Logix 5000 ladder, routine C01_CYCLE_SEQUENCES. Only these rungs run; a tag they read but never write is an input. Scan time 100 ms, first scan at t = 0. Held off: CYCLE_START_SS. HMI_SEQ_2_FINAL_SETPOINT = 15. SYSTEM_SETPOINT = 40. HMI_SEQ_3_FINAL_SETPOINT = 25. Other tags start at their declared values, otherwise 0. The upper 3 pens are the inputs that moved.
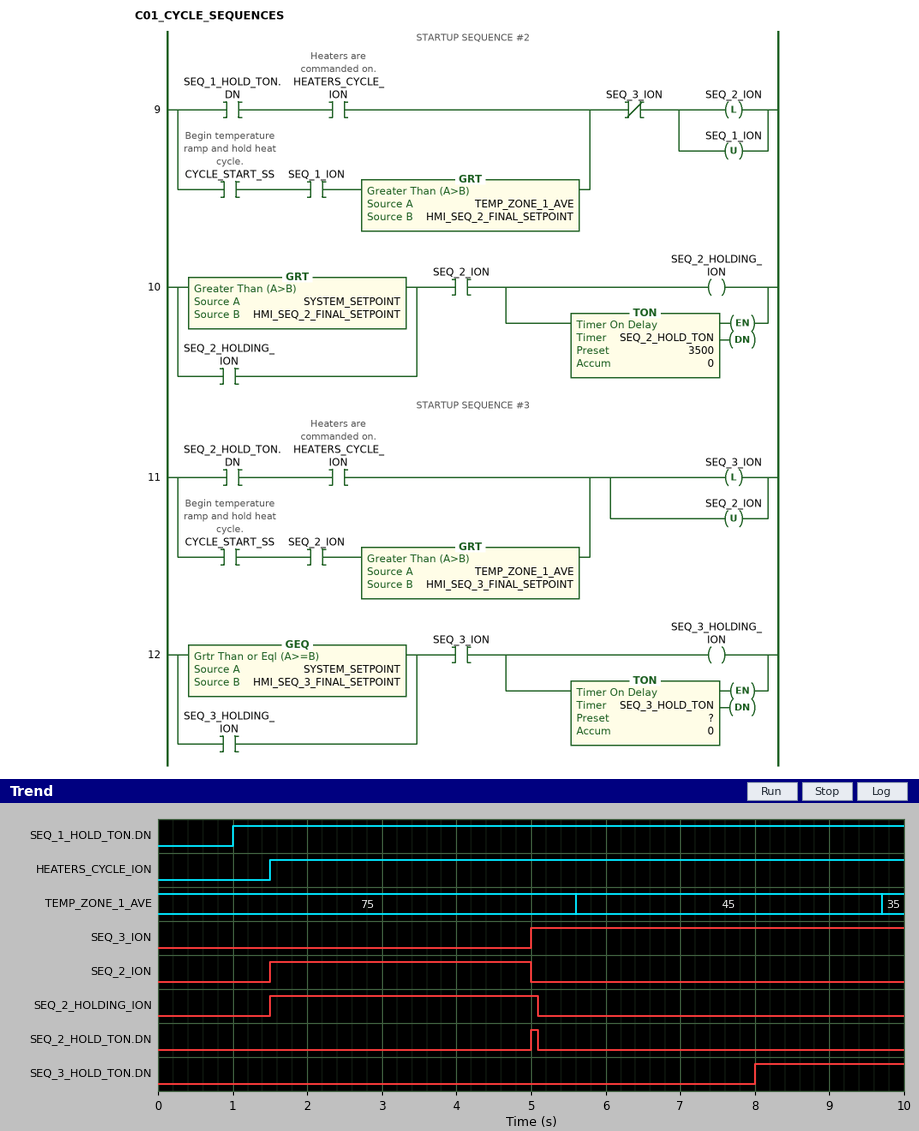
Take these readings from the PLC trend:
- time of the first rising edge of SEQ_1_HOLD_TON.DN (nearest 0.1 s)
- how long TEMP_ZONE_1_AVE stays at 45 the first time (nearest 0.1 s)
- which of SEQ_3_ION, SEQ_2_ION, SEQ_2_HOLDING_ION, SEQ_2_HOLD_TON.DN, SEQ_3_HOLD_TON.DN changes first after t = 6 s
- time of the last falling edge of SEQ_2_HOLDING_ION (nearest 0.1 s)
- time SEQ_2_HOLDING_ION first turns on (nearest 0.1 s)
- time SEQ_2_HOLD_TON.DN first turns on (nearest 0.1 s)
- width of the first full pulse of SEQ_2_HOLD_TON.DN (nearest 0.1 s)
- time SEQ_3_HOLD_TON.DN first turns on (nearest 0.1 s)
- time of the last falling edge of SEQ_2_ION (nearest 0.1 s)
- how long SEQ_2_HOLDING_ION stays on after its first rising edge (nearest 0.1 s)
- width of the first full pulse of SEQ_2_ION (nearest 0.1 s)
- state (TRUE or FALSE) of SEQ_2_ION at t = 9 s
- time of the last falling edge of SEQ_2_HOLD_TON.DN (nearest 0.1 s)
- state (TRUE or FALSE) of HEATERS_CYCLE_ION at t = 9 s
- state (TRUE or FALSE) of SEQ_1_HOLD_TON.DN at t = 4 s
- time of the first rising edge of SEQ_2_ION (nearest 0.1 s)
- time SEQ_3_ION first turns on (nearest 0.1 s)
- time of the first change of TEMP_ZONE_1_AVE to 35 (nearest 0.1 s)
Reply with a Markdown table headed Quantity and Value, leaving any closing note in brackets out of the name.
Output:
| Quantity | Value |
|---|---|
| time of the first rising edge of SEQ_1_HOLD_TON.DN | 1.0 s |
| how long TEMP_ZONE_1_AVE stays at 45 the first time | 4.1 s |
| which of SEQ_3_ION, SEQ_2_ION, SEQ_2_HOLDING_ION, SEQ_2_HOLD_TON.DN, SEQ_3_HOLD_TON.DN changes first after t = 6 s | SEQ_3_HOLD_TON.DN |
| time of the last falling edge of SEQ_2_HOLDING_ION | 5.1 s |
| time SEQ_2_HOLDING_ION first turns on | 1.5 s |
| time SEQ_2_HOLD_TON.DN first turns on | 5.0 s |
| width of the first full pulse of SEQ_2_HOLD_TON.DN | 0.1 s |
| time SEQ_3_HOLD_TON.DN first turns on | 8.0 s |
| time of the last falling edge of SEQ_2_ION | 5.0 s |
| how long SEQ_2_HOLDING_ION stays on after its first rising edge | 3.6 s |
| width of the first full pulse of SEQ_2_ION | 3.5 s |
| state (TRUE or FALSE) of SEQ_2_ION at t = 9 s | FALSE |
| time of the last falling edge of SEQ_2_HOLD_TON.DN | 5.1 s |
| state (TRUE or FALSE) of HEATERS_CYCLE_ION at t = 9 s | TRUE |
| state (TRUE or FALSE) of SEQ_1_HOLD_TON.DN at t = 4 s | TRUE |
| time of the first rising edge of SEQ_2_ION | 1.5 s |
| time SEQ_3_ION first turns on | 5.0 s |
| time of the first change of TEMP_ZONE_1_AVE to 35 | 9.7 s |
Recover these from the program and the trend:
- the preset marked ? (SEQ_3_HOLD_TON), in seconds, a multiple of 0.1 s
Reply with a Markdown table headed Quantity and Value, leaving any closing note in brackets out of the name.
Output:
| Quantity | Value |
|---|---|
| the preset marked ? (SEQ_3_HOLD_TON), in seconds, a multiple of 0.1 s | 3.0 s |
